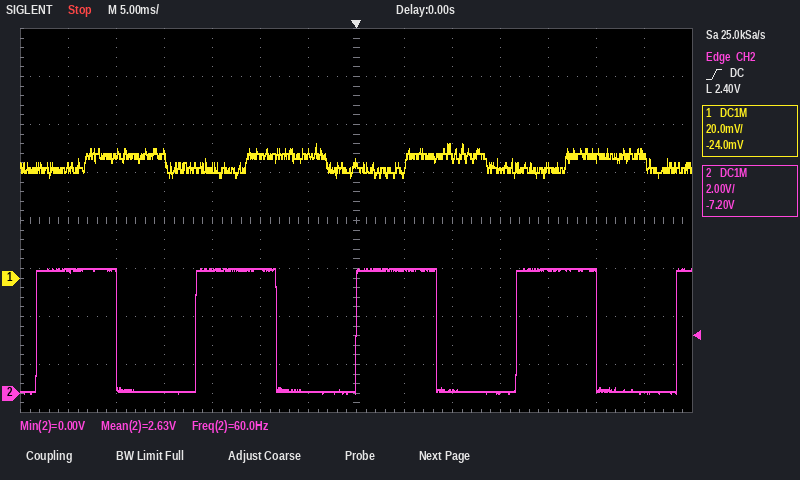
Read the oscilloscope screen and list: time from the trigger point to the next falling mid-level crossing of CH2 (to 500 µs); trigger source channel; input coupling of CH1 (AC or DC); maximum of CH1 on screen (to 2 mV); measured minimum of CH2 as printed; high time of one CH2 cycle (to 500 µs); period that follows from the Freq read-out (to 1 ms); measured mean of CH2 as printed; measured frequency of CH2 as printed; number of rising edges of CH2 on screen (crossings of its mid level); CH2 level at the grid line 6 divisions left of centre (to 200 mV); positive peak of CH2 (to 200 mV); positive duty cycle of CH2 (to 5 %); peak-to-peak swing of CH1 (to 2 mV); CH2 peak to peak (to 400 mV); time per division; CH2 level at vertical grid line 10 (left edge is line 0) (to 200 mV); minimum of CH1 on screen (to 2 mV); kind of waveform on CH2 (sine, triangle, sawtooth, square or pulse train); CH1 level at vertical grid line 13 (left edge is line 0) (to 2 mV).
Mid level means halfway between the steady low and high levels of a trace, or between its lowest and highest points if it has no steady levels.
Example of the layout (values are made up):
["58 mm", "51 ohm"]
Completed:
["8.5 ms", "CH2", "DC", "56 mV", "0.00 V", "8.5 ms", "17 ms", "2.63 V", "60.0 Hz", "5", "5.2 V", "5.2 V", "50 %", "14 mV", "5.2 V", "5 ms", "0.0 V", "42 mV", "square", "52 mV"]
